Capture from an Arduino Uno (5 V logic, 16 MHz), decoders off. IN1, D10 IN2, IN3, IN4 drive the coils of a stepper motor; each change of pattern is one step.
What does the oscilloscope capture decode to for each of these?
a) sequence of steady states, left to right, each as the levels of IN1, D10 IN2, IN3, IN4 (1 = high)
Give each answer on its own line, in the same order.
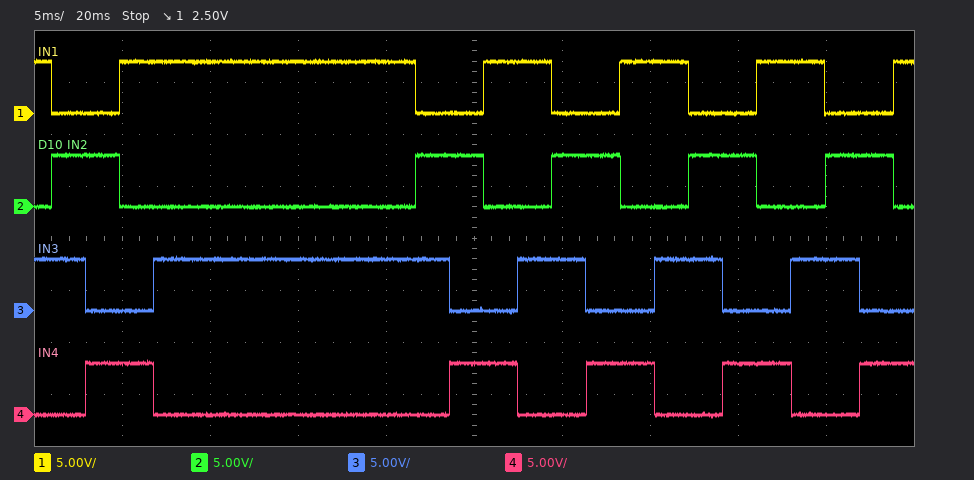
1010 0110 0101 1001 1010 0110 0101 1001 1010 0110 0101 1001 1010 0110 0101 1001 1010 0110 0101 1001
